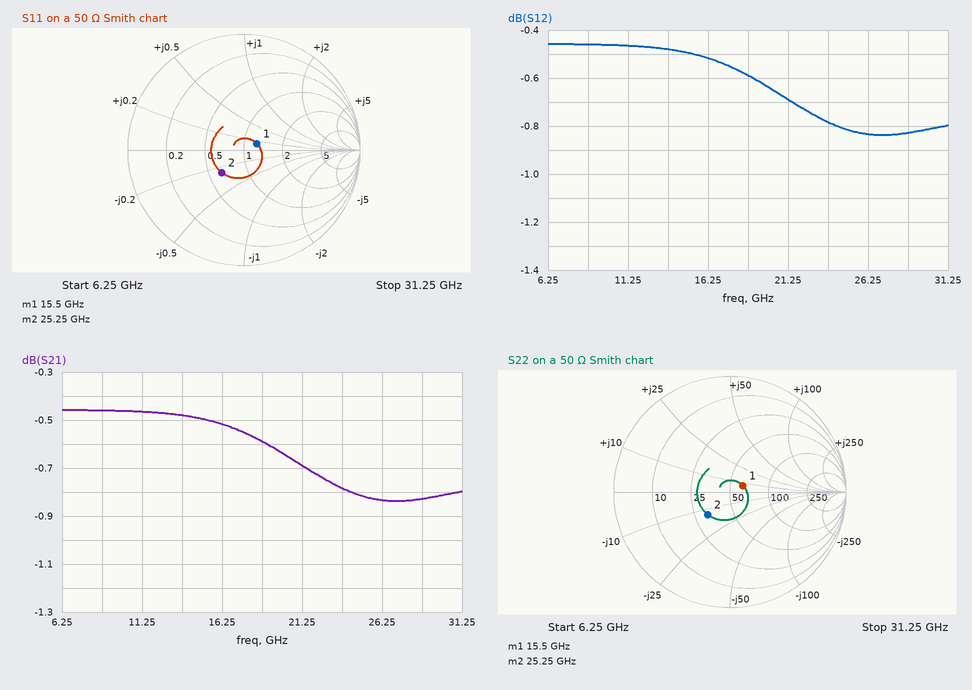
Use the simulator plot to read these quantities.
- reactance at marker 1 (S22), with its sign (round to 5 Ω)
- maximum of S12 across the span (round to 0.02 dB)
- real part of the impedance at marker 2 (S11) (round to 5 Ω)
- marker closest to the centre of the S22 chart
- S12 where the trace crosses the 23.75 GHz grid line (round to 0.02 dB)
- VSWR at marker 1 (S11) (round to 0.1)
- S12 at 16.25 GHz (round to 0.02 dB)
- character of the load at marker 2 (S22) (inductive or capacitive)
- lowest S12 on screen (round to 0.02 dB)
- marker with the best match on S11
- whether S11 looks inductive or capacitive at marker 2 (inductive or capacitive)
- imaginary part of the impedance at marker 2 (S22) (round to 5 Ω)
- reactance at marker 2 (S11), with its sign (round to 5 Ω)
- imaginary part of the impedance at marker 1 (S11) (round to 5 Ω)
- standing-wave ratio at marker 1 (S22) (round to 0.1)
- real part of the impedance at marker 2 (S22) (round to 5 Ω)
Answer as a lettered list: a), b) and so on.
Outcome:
a) +5 Ω
b) -0.46 dB
c) 30 Ω
d) marker 1
e) -0.78 dB
f) 1.3
g) -0.52 dB
h) capacitive
i) -0.84 dB
j) marker 1
k) capacitive
l) -15 Ω
m) -15 Ω
n) +5 Ω
o) 1.3
p) 30 Ω
